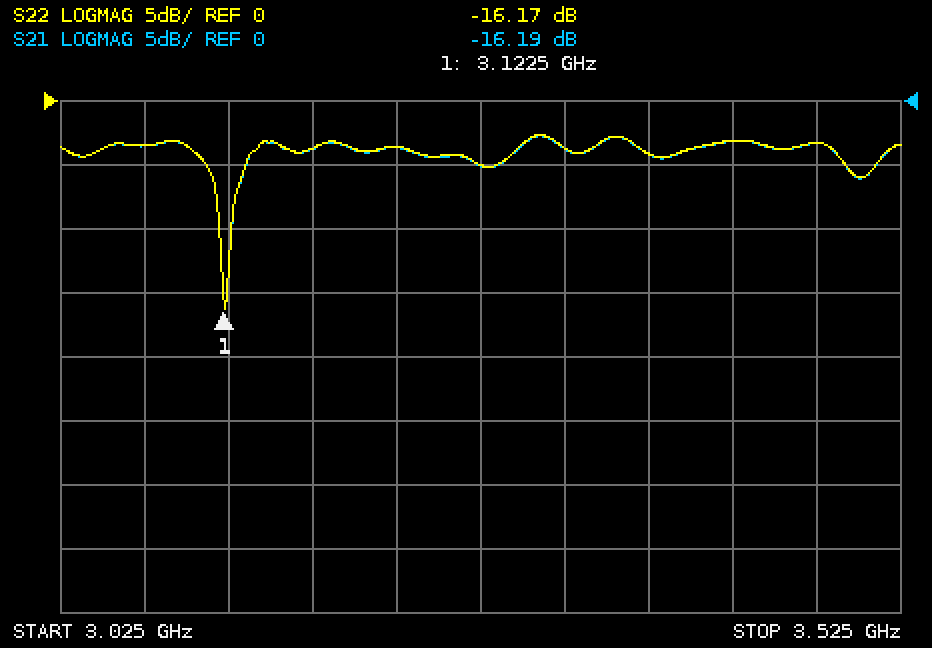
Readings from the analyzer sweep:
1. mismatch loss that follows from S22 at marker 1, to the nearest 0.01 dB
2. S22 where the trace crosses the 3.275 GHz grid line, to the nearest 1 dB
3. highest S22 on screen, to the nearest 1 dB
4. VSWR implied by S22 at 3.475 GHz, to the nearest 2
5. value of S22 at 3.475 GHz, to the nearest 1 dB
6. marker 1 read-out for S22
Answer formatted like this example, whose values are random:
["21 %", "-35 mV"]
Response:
["0.11 dB", "-5 dB", "-3 dB", "6", "-3 dB", "-16.17 dB"]
